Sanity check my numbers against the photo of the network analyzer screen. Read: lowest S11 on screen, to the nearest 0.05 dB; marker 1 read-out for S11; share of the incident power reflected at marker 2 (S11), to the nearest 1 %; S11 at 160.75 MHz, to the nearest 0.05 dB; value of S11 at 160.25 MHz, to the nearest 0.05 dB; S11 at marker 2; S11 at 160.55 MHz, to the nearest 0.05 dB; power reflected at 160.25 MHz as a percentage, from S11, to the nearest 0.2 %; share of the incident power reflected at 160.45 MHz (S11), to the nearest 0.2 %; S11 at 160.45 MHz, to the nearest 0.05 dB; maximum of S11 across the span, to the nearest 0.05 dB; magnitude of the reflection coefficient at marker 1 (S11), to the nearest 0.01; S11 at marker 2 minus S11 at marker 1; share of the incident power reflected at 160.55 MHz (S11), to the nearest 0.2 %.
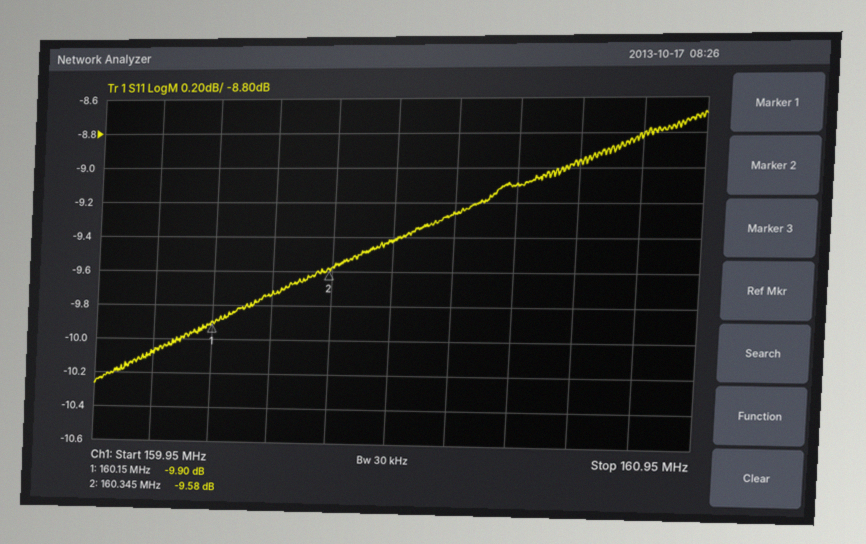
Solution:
-10.25 dB
-9.90 dB
11 %
-8.95 dB
-9.75 dB
-9.58 dB
-9.25 dB
10.6 %
11.4 %
-9.40 dB
-8.70 dB
0.32
0.32 dB
11.8 %
